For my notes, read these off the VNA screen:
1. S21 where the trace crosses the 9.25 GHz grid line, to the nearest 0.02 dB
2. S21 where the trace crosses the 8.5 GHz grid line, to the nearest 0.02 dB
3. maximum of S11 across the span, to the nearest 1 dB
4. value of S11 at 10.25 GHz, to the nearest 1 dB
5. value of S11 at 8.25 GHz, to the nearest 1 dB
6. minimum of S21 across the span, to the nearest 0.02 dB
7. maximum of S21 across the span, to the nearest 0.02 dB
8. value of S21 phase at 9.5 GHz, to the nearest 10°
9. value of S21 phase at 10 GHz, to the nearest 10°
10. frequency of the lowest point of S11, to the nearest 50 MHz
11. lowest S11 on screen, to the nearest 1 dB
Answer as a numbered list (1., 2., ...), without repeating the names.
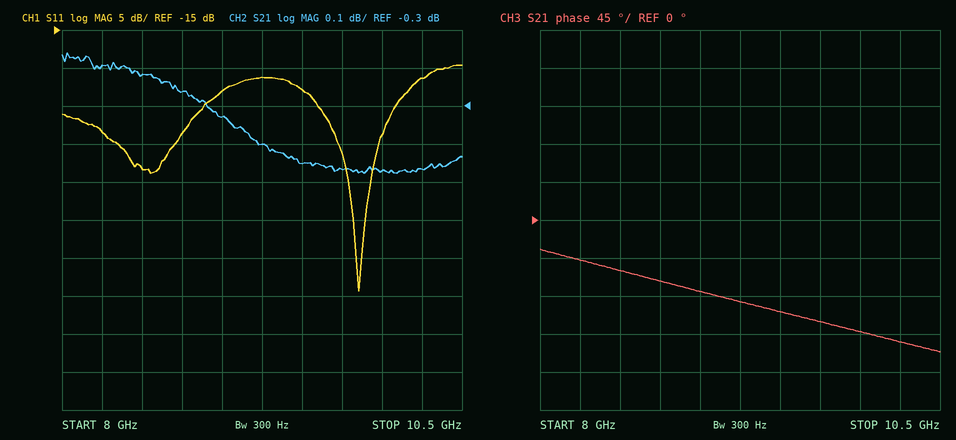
1. -0.40 dB
2. -0.22 dB
3. -20 dB
4. -21 dB
5. -28 dB
6. -0.48 dB
7. -0.16 dB
8. -110°
9. -130°
10. 9.85 GHz
11. -49 dB
